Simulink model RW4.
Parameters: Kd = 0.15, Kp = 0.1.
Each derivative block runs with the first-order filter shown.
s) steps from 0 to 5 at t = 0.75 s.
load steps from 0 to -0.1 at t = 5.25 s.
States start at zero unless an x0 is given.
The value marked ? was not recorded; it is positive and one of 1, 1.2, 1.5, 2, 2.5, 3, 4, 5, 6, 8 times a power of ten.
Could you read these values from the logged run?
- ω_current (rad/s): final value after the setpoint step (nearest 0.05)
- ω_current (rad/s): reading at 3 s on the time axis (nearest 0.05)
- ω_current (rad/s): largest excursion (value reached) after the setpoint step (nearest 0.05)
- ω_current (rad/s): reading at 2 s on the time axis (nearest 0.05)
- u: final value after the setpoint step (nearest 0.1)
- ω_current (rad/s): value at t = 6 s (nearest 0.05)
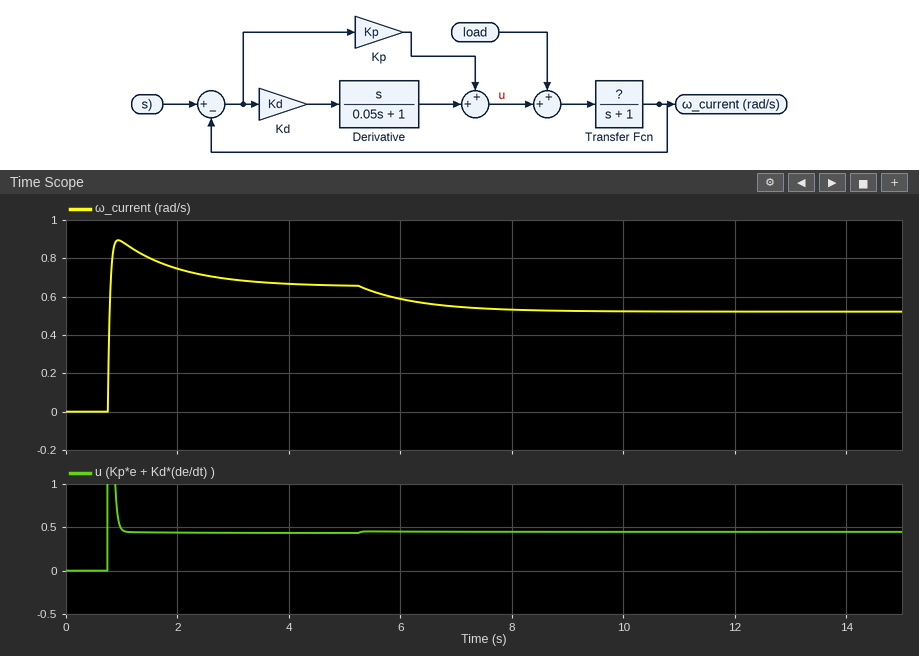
0.65
0.70
0.90
0.75
0.4
0.60
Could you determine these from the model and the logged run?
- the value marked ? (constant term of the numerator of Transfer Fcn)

1.5
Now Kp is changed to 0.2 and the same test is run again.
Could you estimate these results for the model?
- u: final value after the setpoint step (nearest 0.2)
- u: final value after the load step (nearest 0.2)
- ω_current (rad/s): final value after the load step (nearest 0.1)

0.8
0.8
1.0
